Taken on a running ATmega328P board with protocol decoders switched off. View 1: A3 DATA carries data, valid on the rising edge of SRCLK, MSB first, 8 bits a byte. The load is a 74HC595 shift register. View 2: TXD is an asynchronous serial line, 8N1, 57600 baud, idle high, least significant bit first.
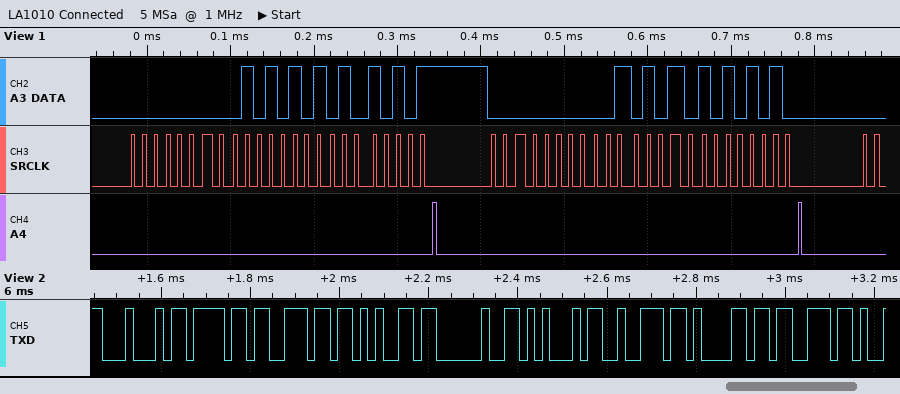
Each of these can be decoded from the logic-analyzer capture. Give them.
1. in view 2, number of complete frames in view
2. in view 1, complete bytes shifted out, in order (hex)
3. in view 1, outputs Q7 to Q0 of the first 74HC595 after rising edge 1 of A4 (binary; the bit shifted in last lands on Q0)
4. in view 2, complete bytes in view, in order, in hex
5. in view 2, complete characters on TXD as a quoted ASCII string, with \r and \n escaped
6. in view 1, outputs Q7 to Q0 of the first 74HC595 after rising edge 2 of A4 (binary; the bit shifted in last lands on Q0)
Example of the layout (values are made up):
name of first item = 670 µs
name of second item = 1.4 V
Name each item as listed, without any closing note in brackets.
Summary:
in view 2, number of complete frames in view = 9
in view 1, complete bytes shifted out, in order = 00 55 55 00 2A AA
in view 1, outputs Q7 to Q0 of the first 74HC595 after rising edge 1 of A4 = 01010101
in view 2, complete bytes in view, in order, in hex = 44 6F 6E 65 20 45 72 61 73
in view 2, complete characters on TXD as a quoted ASCII string, with \r and \n escaped = "Done Eras"
in view 1, outputs Q7 to Q0 of the first 74HC595 after rising edge 2 of A4 = 10101010
